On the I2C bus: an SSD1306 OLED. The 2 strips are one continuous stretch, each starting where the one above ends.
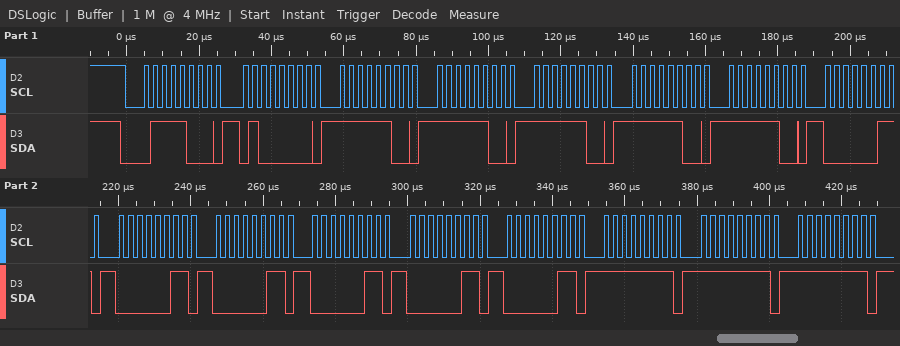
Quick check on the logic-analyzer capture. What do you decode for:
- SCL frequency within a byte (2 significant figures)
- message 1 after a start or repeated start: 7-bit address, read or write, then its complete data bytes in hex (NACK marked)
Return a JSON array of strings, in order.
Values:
["400 kHz", "0x3C write: 40 FC FC FC FC FC 03 03 03 03 03 03 FF FF FF"]
